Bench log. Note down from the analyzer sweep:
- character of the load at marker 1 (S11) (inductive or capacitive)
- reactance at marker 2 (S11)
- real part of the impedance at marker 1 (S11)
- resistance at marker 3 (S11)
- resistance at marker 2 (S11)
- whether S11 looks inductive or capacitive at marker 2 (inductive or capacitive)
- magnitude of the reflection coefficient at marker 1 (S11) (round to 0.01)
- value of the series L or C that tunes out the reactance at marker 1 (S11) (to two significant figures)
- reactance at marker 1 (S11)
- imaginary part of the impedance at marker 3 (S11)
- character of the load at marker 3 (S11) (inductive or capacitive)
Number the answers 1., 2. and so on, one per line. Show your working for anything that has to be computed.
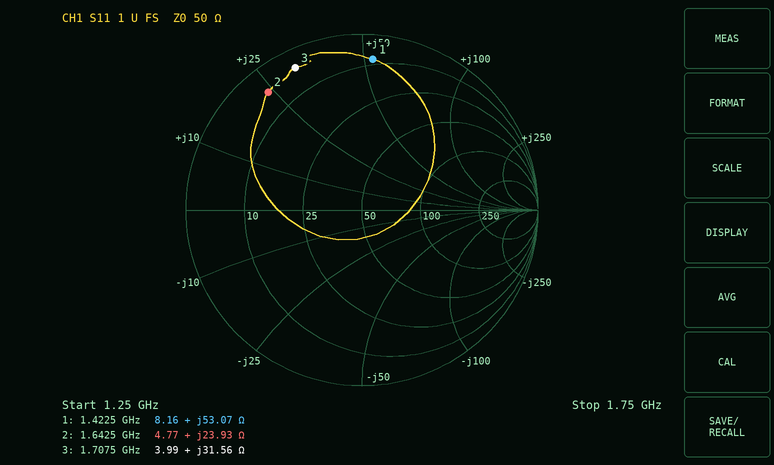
1. inductive
2. +23.93 Ω
3. 8.16 Ω
4. 3.99 Ω
5. 4.77 Ω
6. inductive
7. 0.86
8. C = 1/(2π × 1.4225 GHz × 53.07 Ω) ≈ 2.1 pF
9. +53.07 Ω
10. +31.56 Ω
11. inductive
